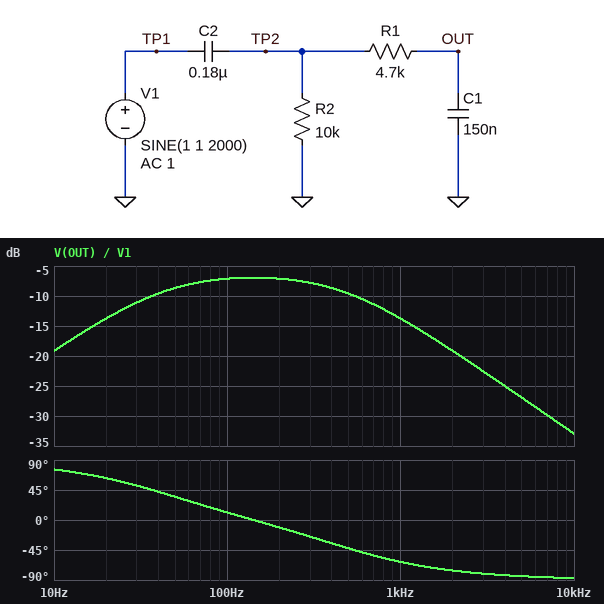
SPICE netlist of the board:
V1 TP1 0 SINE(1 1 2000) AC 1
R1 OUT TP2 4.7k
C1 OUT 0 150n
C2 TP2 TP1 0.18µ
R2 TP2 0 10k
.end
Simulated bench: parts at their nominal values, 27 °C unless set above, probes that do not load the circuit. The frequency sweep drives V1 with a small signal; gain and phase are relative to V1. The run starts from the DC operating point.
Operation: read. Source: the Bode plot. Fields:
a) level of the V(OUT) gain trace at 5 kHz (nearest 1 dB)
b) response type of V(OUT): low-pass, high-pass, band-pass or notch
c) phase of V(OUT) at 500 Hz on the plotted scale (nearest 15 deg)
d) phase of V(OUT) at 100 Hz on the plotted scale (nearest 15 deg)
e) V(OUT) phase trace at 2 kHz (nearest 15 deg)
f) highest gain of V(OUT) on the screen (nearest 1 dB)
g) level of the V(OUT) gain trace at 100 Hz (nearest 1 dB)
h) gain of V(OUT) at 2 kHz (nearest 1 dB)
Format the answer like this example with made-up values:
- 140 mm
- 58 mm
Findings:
- -27 dB
- band-pass
- -45 deg
- 15 deg
- -75 deg
- -7 dB
- -7 dB
- -19 dB
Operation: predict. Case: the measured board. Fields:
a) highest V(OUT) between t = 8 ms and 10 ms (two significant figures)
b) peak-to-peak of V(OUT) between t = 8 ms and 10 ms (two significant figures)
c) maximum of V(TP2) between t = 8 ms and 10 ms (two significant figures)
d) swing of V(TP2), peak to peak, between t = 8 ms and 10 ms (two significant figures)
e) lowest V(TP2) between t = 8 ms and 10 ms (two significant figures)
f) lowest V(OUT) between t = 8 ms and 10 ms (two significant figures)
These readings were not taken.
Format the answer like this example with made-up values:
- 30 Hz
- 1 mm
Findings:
- 110 mV
- 220 mV
- 980 mV
- 2.0 V
- -980 mV
- -110 mV
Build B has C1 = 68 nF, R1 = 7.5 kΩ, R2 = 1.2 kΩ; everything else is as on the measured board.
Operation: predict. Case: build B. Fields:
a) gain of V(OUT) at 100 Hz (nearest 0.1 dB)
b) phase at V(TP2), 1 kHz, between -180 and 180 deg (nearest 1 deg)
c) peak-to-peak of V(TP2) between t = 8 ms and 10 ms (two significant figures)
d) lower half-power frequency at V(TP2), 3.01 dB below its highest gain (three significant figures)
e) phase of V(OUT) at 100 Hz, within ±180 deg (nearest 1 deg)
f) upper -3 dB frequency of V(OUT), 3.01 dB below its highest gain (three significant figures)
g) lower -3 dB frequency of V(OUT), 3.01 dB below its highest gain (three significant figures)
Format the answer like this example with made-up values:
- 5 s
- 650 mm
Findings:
- -18.0 dB
- 39 deg
- 1.8 V
- 880 Hz
- 62 deg
- 1.34 kHz
- 172 Hz
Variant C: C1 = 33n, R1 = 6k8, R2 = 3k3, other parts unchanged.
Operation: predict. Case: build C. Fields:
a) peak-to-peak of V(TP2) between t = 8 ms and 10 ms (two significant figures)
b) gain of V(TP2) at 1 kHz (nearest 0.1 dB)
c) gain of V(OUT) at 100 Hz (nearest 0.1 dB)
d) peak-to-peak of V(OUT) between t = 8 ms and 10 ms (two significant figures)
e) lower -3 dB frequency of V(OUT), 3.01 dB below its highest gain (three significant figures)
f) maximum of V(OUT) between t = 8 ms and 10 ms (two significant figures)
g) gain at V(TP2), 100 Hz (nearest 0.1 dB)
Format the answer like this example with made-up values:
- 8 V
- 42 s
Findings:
- 1.9 V
- -1.0 dB
- -9.5 dB
- 640 mV
- 151 Hz
- 320 mV
- -9.4 dB
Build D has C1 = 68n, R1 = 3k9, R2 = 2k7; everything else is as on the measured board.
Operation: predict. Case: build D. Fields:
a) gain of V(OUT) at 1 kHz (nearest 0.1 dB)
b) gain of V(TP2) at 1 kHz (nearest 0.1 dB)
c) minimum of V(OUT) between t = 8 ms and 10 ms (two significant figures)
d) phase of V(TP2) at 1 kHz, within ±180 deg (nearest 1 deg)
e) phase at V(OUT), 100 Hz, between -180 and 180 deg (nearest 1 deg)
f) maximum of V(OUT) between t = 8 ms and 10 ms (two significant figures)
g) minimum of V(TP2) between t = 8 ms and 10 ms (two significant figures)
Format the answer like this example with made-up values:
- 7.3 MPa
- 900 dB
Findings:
- -7.4 dB
- -1.6 dB
- -270 mV
- 24 deg
- 58 deg
- 270 mV
- -940 mV
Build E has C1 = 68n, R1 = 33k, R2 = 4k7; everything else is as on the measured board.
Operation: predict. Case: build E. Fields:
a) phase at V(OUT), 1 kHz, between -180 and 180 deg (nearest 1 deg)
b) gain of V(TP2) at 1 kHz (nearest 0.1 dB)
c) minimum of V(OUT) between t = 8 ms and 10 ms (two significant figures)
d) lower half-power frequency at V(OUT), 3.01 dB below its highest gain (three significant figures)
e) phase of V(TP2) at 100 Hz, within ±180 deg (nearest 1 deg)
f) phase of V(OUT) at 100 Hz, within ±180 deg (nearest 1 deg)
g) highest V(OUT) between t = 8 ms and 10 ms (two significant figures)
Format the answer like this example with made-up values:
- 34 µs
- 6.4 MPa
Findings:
- -74 deg
- -0.2 dB
- -36 mV
- 40.8 Hz
- 61 deg
- 7 deg
- 35 mV
